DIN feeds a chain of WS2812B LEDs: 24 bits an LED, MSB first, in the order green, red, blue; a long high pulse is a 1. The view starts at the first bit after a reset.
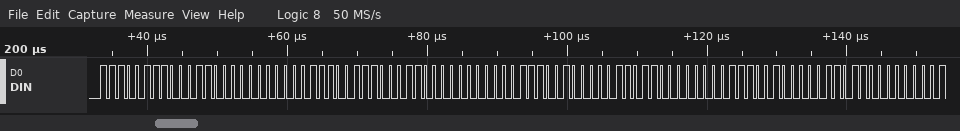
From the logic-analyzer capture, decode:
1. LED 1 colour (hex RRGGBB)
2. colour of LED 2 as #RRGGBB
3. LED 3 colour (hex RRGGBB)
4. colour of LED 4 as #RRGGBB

#18E700
#18E700
#1BE400
#1BE400
